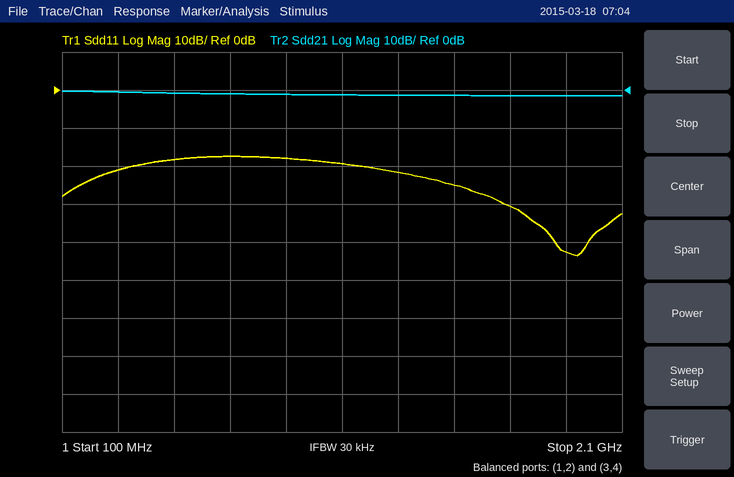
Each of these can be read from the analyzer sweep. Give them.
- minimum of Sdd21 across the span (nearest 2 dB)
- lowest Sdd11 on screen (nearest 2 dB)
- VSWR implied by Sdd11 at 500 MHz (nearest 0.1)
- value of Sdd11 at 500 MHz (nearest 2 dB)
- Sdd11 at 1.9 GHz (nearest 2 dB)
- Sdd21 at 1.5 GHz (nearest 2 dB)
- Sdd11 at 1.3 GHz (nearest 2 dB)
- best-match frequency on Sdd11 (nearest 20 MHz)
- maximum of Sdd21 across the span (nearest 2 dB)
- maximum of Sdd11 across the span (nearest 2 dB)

-2 dB
-44 dB
1.3
-18 dB
-42 dB
-2 dB
-22 dB
1.94 GHz
0 dB
-18 dB
